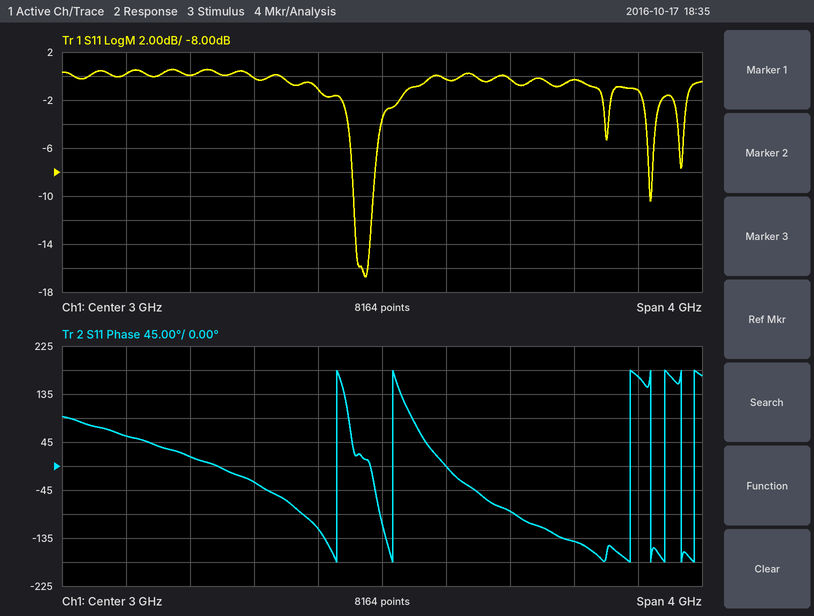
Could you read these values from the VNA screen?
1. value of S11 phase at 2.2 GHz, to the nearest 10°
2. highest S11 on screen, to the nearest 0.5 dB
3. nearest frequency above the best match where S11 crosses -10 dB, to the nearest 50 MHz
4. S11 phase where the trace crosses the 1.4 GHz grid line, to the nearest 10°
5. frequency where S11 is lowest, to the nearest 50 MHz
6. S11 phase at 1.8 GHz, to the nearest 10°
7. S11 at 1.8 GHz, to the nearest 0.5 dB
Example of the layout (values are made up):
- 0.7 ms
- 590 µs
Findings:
- -30°
- 0.5 dB
- 2.95 GHz
- 60°
- 2.90 GHz
- 20°
- 0.0 dB
